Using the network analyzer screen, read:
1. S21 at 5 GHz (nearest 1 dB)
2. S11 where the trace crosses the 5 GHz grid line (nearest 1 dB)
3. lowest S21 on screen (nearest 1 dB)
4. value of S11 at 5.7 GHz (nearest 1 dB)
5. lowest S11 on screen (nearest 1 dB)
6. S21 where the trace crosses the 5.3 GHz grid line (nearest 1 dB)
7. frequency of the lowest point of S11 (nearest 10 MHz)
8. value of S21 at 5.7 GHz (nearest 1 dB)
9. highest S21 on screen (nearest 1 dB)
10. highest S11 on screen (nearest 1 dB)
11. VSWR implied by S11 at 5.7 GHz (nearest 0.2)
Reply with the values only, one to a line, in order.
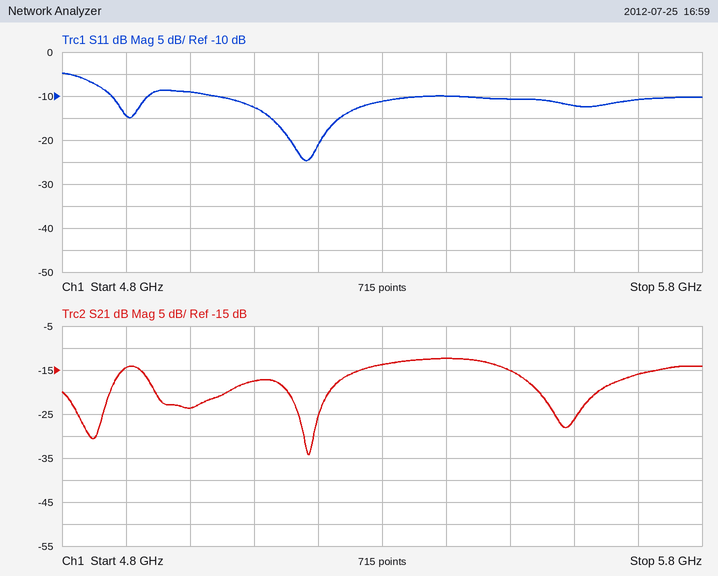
-24 dB
-9 dB
-34 dB
-11 dB
-25 dB
-14 dB
5.18 GHz
-16 dB
-12 dB
-5 dB
1.8
